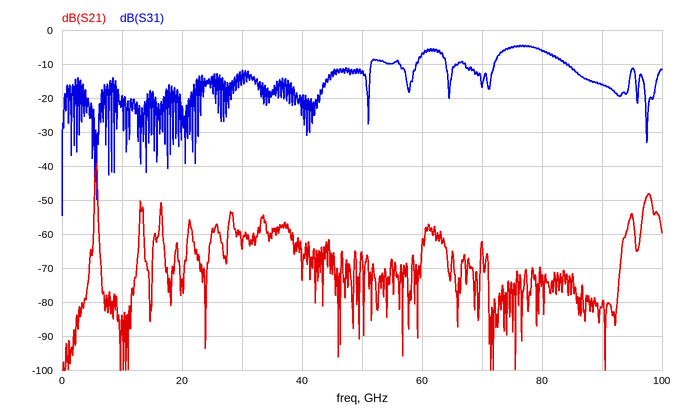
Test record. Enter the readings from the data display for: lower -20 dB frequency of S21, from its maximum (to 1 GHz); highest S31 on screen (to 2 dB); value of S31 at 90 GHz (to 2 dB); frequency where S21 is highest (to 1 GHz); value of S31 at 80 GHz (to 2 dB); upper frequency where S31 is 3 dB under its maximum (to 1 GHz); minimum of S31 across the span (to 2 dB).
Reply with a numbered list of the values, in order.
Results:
1. 5 GHz
2. -4 dB
3. -16 dB
4. 6 GHz
5. -6 dB
6. 82 GHz
7. -54 dB
